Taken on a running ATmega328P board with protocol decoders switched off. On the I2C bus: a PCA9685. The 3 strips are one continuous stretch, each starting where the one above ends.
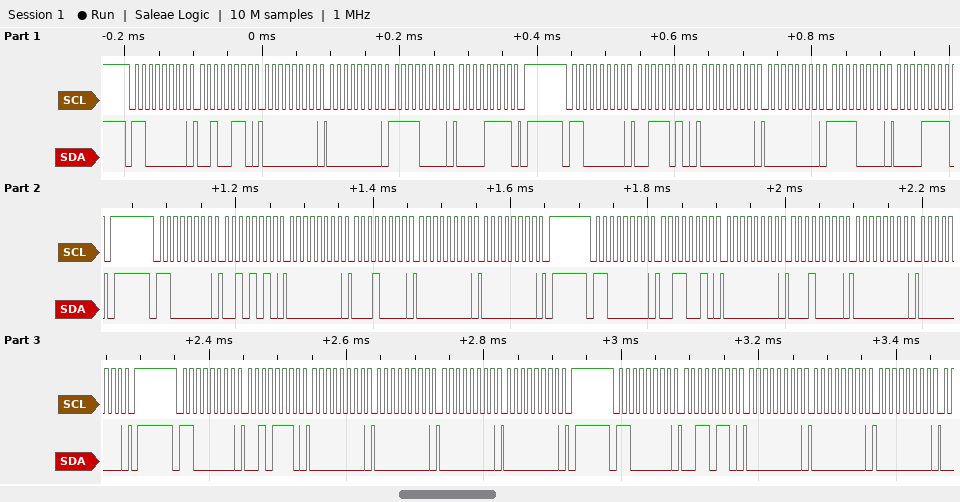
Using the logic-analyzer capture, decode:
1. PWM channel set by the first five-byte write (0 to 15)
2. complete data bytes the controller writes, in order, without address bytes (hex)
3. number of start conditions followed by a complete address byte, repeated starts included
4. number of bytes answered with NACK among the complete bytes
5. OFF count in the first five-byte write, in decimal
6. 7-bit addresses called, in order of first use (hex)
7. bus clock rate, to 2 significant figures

8
26 00 00 F0 0F 3A 00 00 F0 0F 2A 00 10 00 00 32 00 10 00 00 2E 00 00 00 00 36 00 00 00
6
0
4080
0x60
100 kHz
